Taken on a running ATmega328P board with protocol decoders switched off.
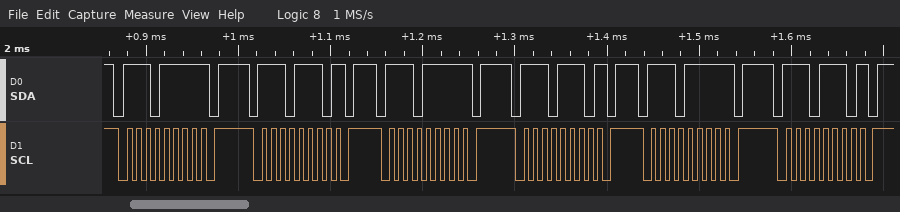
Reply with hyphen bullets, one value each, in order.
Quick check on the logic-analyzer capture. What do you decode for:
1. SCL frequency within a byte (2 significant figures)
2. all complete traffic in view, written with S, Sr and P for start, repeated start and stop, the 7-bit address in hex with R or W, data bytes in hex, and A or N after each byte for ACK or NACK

- 100 kHz
- S 77R N P S 77W N P S 77R N P S 77W N P S 77R N P S 77W N P
